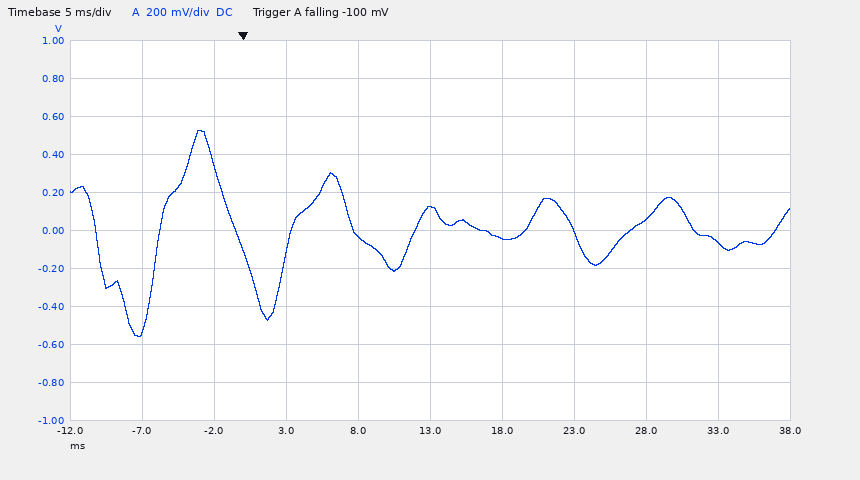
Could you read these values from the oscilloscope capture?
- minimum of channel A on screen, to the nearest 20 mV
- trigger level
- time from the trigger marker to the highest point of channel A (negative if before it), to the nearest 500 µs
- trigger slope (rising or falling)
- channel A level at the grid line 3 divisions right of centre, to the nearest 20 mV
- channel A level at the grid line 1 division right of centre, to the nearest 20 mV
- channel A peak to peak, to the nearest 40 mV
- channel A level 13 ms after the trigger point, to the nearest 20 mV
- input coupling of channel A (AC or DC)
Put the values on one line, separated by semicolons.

-560 mV; -100 mV; -3.0 ms; falling; 60 mV; -40 mV; 1.08 V; 120 mV; DC
